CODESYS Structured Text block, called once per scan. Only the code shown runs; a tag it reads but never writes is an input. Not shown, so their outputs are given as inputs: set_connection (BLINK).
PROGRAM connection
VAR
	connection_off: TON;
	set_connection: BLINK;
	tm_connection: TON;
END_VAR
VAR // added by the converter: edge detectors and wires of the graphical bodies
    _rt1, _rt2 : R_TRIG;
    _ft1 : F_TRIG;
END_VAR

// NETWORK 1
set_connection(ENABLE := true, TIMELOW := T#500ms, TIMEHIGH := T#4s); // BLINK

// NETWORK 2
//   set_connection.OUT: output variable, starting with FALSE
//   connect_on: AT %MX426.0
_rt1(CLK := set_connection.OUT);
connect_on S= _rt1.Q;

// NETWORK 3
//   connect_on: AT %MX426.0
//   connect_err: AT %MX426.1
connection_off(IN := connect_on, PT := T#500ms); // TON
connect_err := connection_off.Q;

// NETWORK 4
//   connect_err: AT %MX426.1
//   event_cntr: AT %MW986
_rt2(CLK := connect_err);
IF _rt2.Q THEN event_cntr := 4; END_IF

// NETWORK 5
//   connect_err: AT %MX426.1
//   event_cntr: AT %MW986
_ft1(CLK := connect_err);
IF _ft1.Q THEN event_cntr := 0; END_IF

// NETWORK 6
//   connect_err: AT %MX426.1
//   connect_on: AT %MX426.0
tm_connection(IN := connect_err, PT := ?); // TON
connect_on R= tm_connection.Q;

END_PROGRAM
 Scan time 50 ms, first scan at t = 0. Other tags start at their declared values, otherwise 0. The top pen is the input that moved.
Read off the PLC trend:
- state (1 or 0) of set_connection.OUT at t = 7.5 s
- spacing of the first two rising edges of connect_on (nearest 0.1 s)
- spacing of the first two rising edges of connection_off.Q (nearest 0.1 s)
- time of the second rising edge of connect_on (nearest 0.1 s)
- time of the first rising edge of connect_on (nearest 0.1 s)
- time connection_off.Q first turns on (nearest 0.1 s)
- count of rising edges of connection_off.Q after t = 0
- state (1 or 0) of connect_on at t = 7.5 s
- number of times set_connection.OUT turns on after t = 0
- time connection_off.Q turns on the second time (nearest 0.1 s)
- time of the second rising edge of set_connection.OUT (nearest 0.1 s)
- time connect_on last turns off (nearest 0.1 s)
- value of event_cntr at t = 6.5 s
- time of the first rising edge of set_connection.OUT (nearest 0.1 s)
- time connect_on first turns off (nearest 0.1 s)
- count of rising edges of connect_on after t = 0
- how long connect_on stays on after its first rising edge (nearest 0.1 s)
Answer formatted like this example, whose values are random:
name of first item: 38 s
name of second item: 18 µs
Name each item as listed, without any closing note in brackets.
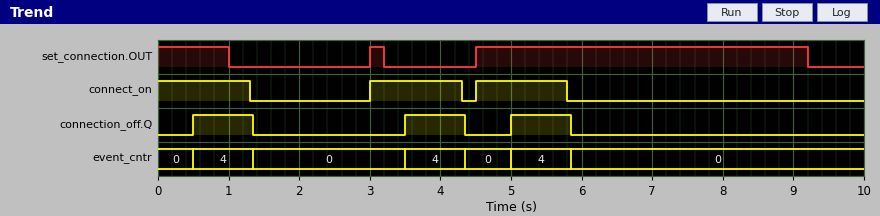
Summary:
state (1 or 0) of set_connection.OUT at t = 7.5 s: 1
spacing of the first two rising edges of connect_on: 1.5 s
spacing of the first two rising edges of connection_off.Q: 3.0 s
time of the second rising edge of connect_on: 4.5 s
time of the first rising edge of connect_on: 3.0 s
time connection_off.Q first turns on: 0.5 s
count of rising edges of connection_off.Q after t = 0: 3
state (1 or 0) of connect_on at t = 7.5 s: 0
number of times set_connection.OUT turns on after t = 0: 2
time connection_off.Q turns on the second time: 3.5 s
time of the second rising edge of set_connection.OUT: 4.5 s
time connect_on last turns off: 5.8 s
value of event_cntr at t = 6.5 s: 0
time of the first rising edge of set_connection.OUT: 3.0 s
time connect_on first turns off: 1.3 s
count of rising edges of connect_on after t = 0: 2
how long connect_on stays on after its first rising edge: 1.3 s
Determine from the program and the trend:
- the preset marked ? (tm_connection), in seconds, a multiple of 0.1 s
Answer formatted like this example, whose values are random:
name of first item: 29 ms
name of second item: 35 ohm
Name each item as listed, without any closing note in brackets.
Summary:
the preset marked ? (tm_connection), in seconds, a multiple of 0.1 s: 0.8 s
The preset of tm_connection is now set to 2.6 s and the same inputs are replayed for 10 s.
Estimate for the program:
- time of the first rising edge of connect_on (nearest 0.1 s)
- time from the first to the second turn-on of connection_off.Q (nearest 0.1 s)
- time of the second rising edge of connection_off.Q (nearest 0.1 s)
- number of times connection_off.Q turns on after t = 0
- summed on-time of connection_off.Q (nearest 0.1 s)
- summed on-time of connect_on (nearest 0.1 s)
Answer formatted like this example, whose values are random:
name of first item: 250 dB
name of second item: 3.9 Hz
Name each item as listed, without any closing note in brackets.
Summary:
time of the first rising edge of connect_on: 4.5 s
time from the first to the second turn-on of connection_off.Q: 4.5 s
time of the second rising edge of connection_off.Q: 5.0 s
number of times connection_off.Q turns on after t = 0: 2
summed on-time of connection_off.Q: 5.3 s
summed on-time of connect_on: 6.2 s
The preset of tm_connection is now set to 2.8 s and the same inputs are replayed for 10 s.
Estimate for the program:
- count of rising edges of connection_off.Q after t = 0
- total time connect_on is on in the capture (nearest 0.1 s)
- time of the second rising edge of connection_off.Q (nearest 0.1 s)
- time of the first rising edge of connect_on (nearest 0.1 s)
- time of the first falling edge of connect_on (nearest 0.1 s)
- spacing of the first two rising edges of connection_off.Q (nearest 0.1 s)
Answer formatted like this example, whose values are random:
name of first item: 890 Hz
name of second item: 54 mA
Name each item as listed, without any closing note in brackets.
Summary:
count of rising edges of connection_off.Q after t = 0: 2
total time connect_on is on in the capture: 6.6 s
time of the second rising edge of connection_off.Q: 5.0 s
time of the first rising edge of connect_on: 4.5 s
time of the first falling edge of connect_on: 3.3 s
spacing of the first two rising edges of connection_off.Q: 4.5 s
